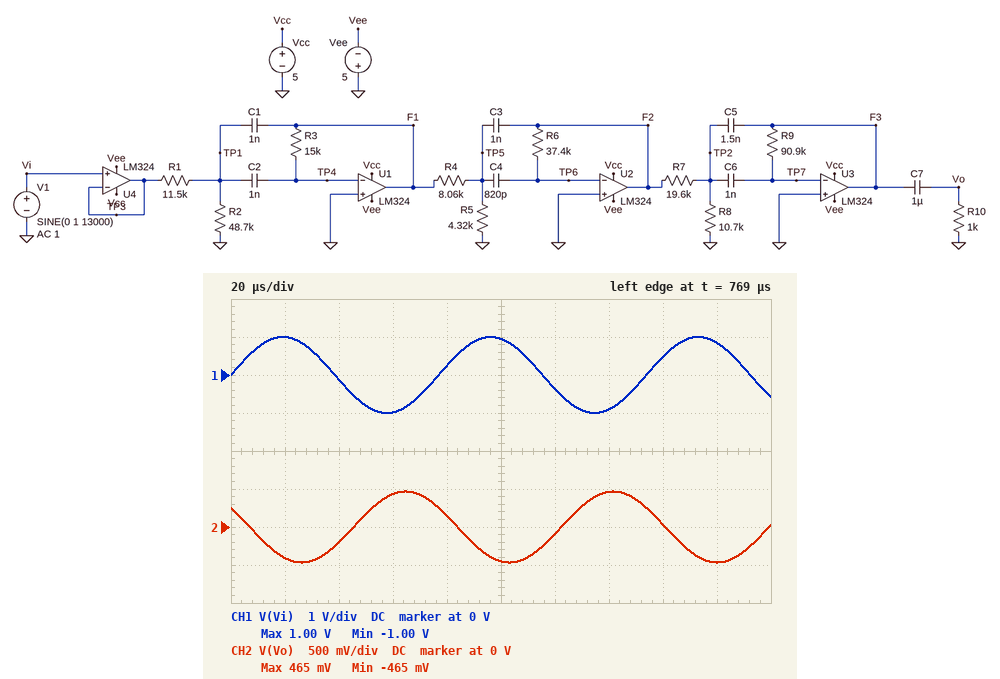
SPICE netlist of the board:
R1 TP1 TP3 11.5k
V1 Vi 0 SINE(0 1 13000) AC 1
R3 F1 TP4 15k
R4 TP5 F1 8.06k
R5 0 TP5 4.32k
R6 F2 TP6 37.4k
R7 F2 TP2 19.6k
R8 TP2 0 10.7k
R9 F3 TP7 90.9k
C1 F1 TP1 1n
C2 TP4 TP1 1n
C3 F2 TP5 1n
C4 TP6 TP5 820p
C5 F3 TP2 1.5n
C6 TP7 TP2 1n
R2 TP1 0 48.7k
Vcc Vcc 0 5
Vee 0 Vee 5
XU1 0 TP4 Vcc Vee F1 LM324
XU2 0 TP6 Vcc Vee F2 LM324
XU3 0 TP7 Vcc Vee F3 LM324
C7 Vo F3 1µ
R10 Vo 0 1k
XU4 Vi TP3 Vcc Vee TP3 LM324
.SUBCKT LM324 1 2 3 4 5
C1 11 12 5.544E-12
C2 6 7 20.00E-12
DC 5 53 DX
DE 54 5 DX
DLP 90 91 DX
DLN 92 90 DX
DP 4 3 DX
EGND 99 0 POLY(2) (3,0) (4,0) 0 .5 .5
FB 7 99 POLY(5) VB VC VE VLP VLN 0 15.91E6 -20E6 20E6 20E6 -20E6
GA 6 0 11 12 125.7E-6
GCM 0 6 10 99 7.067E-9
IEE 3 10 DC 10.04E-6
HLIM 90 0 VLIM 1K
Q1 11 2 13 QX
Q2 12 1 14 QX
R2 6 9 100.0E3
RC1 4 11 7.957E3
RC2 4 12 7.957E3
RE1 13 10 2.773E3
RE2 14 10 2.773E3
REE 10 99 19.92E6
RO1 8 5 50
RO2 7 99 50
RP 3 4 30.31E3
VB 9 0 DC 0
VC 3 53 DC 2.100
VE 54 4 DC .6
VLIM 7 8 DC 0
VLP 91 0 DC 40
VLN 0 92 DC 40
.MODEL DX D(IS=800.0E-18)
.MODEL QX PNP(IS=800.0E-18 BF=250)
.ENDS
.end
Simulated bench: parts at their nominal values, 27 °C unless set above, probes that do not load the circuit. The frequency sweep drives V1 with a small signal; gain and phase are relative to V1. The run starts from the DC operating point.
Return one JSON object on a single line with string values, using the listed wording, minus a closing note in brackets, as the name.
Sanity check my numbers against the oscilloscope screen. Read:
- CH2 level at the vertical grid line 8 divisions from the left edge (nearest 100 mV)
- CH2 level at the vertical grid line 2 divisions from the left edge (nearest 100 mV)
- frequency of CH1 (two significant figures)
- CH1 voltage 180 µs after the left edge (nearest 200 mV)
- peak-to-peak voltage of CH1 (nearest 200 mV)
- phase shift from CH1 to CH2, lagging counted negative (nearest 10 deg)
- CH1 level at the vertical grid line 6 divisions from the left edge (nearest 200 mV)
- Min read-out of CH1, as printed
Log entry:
{"CH2 level at the vertical grid line 8 divisions from the left edge": "0 V", "CH2 level at the vertical grid line 2 divisions from the left edge": "-200 mV", "frequency of CH1": "13 kHz", "CH1 voltage 180 µs after the left edge": "800 mV", "peak-to-peak voltage of CH1": "2.0 V", "phase shift from CH1 to CH2, lagging counted negative": "150 deg", "CH1 level at the vertical grid line 6 divisions from the left edge": "-400 mV", "Min read-out of CH1, as printed": "-1.00 V"}
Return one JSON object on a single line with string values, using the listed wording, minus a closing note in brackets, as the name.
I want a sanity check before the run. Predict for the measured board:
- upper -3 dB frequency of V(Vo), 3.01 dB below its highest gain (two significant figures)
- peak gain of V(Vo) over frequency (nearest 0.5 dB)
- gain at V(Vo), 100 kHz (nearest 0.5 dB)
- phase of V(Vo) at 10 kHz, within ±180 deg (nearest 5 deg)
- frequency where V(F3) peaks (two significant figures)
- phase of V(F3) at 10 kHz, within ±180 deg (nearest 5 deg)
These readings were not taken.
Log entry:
{"upper -3 dB frequency of V(Vo), 3.01 dB below its highest gain": "19 kHz", "peak gain of V(Vo) over frequency": "-6.0 dB", "gain at V(Vo), 100 kHz": "-57.0 dB", "phase of V(Vo) at 10 kHz, within ±180 deg": "-165 deg", "frequency where V(F3) peaks": "15 kHz", "phase of V(F3) at 10 kHz, within ±180 deg": "-165 deg"}
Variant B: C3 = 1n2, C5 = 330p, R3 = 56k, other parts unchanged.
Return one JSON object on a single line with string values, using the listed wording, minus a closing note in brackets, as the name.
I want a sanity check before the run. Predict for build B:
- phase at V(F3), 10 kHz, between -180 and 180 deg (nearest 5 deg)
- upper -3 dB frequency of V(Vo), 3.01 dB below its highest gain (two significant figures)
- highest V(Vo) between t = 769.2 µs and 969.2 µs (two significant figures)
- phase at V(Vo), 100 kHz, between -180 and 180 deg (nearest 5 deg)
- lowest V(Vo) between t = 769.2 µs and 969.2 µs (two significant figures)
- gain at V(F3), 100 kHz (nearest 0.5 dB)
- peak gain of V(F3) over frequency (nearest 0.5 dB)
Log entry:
{"phase at V(F3), 10 kHz, between -180 and 180 deg": "-155 deg", "upper -3 dB frequency of V(Vo), 3.01 dB below its highest gain": "15 kHz", "highest V(Vo) between t = 769.2 µs and 969.2 µs": "3.6 V", "phase at V(Vo), 100 kHz, between -180 and 180 deg": "-100 deg", "lowest V(Vo) between t = 769.2 µs and 969.2 µs": "-4.7 V", "gain at V(F3), 100 kHz": "-46.0 dB", "peak gain of V(F3) over frequency": "16.0 dB"}
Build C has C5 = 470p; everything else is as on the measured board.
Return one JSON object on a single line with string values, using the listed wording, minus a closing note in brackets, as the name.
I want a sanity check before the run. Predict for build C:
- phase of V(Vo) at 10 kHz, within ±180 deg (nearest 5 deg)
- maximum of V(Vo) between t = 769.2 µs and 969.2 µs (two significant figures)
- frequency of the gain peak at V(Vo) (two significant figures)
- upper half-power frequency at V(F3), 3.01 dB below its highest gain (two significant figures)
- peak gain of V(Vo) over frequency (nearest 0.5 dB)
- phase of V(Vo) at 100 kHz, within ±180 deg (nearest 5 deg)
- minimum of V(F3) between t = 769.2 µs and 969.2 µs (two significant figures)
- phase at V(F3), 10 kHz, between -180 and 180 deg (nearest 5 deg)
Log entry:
{"phase of V(Vo) at 10 kHz, within ±180 deg": "-115 deg", "maximum of V(Vo) between t = 769.2 µs and 969.2 µs": "1.9 V", "frequency of the gain peak at V(Vo)": "14 kHz", "upper half-power frequency at V(F3), 3.01 dB below its highest gain": "18 kHz", "peak gain of V(Vo) over frequency": "5.5 dB", "phase of V(Vo) at 100 kHz, within ±180 deg": "-95 deg", "minimum of V(F3) between t = 769.2 µs and 969.2 µs": "-1.9 V", "phase at V(F3), 10 kHz, between -180 and 180 deg": "-120 deg"}
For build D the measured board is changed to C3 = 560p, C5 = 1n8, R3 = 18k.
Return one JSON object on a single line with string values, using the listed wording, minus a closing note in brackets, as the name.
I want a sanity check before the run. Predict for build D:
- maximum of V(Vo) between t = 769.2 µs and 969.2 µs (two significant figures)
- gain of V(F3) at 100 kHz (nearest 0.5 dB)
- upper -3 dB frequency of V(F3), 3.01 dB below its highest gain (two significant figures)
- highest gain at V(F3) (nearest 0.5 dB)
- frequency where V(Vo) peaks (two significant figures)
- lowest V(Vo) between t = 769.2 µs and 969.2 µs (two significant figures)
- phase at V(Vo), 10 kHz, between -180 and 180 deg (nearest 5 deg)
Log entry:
{"maximum of V(Vo) between t = 769.2 µs and 969.2 µs": "360 mV", "gain of V(F3) at 100 kHz": "-54.0 dB", "upper -3 dB frequency of V(F3), 3.01 dB below its highest gain": "24 kHz", "highest gain at V(F3)": "-8.0 dB", "frequency where V(Vo) peaks": "18 kHz", "lowest V(Vo) between t = 769.2 µs and 969.2 µs": "-360 mV", "phase at V(Vo), 10 kHz, between -180 and 180 deg": "-165 deg"}
